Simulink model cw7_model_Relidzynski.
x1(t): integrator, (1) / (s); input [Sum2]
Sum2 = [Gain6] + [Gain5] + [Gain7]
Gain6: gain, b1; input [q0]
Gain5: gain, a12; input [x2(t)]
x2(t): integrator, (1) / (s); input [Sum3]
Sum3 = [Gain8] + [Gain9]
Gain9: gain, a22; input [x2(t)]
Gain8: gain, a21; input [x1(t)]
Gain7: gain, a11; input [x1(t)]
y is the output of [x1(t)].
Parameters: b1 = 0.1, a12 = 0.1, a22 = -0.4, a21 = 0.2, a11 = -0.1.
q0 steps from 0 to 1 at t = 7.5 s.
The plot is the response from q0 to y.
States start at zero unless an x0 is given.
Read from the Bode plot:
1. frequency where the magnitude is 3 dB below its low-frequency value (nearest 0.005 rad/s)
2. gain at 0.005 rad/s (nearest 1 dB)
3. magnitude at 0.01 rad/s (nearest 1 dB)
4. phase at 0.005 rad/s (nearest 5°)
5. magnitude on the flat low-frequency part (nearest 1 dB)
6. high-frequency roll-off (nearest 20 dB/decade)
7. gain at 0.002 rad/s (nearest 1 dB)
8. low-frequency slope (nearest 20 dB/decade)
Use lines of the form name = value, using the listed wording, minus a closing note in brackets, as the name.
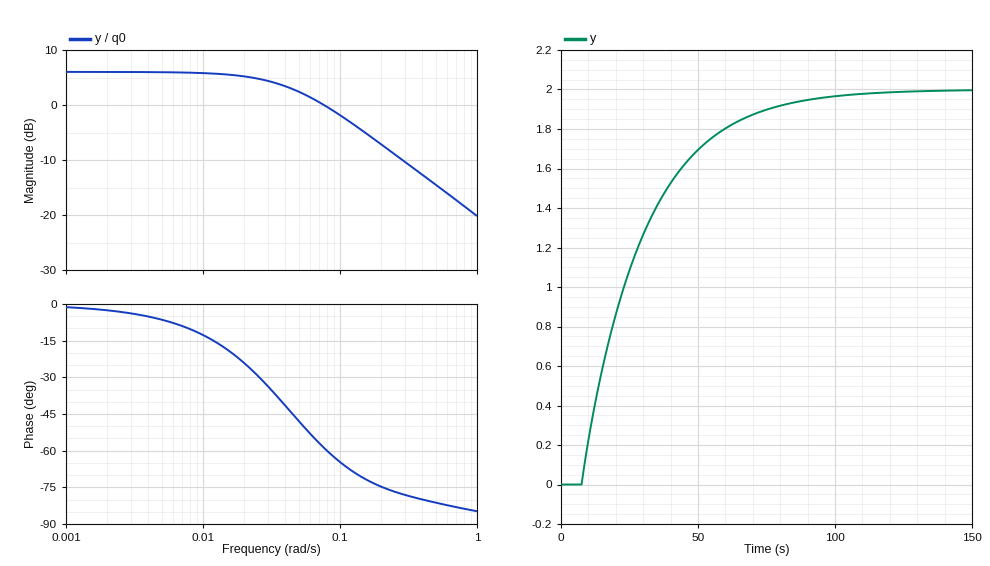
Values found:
frequency where the magnitude is 3 dB below its low-frequency value = 0.045 rad/s
gain at 0.005 rad/s = 6 dB
magnitude at 0.01 rad/s = 6 dB
phase at 0.005 rad/s = -5°
magnitude on the flat low-frequency part = 6 dB
high-frequency roll-off = -20 dB/decade
gain at 0.002 rad/s = 6 dB
low-frequency slope = 0 dB/decade
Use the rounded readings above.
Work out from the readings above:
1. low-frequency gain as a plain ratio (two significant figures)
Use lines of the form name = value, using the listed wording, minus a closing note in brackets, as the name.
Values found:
low-frequency gain as a plain ratio = 2.0
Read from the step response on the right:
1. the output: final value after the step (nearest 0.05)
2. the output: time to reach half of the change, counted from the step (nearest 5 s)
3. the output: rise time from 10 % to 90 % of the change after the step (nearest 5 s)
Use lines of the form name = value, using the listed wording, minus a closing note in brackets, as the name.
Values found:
the output: final value after the step = 2.00
the output: time to reach half of the change, counted from the step = 15 s
the output: rise time from 10 % to 90 % of the change after the step = 50 s
